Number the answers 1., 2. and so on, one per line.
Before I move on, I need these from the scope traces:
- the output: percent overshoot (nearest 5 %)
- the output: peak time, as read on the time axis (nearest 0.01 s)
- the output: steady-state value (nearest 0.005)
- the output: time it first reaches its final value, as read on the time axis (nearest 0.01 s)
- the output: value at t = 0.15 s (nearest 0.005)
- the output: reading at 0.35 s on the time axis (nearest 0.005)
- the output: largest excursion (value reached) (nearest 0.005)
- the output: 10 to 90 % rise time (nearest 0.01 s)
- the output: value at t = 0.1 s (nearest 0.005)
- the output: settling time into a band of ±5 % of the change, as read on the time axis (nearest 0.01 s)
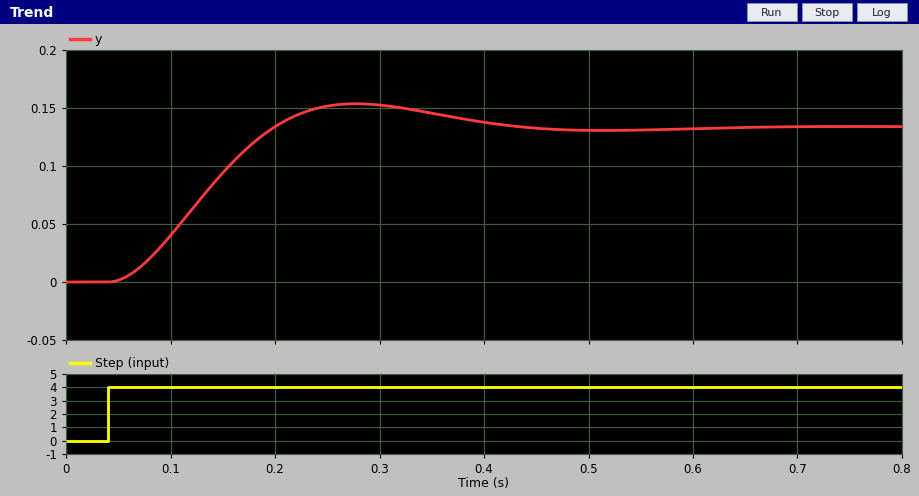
1. 15 %
2. 0.28 s
3. 0.135
4. 0.20 s
5. 0.095
6. 0.145
7. 0.155
8. 0.11 s
9. 0.040
10. 0.38 s
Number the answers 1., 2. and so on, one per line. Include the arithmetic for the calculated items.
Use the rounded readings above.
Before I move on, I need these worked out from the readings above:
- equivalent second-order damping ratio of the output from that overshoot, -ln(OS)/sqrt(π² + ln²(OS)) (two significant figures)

1. ln(0.15) = -1.897; 1.897 / sqrt(9.870 + 3.599) = 0.52
